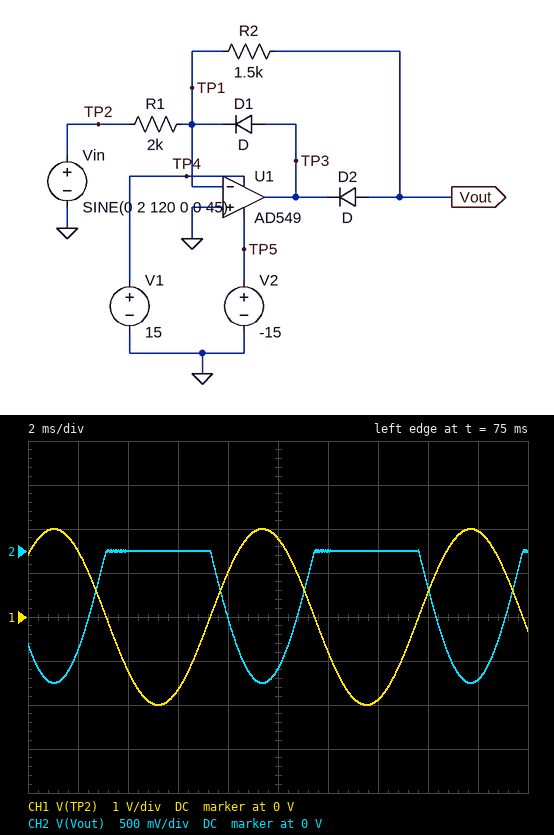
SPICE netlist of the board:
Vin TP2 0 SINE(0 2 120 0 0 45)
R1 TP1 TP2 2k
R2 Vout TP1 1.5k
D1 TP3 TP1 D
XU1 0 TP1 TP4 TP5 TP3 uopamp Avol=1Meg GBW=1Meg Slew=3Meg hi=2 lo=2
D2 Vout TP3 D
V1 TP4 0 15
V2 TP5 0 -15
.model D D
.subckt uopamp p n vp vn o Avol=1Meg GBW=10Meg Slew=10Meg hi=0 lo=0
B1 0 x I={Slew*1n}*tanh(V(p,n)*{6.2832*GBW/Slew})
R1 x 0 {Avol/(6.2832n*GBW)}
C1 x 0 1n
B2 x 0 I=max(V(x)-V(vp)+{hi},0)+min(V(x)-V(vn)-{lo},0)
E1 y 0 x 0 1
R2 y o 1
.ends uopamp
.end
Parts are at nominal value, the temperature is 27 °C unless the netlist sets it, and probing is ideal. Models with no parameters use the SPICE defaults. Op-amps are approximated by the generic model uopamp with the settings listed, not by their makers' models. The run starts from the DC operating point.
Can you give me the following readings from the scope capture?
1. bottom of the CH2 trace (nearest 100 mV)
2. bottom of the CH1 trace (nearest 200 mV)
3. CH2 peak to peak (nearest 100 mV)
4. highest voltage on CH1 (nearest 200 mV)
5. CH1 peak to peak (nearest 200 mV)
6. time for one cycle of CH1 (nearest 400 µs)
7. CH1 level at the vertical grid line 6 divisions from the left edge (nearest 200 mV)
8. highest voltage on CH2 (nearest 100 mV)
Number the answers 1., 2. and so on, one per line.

1. -1.5 V
2. -2.0 V
3. 1.5 V
4. 2.0 V
5. 4.0 V
6. 8.4 ms
7. -800 mV
8. 0 V
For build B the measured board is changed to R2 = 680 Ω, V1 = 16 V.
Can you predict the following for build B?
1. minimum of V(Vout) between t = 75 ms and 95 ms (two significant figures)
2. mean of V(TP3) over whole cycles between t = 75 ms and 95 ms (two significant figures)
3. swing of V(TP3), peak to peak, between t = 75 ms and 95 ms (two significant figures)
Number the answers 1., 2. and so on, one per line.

1. -680 mV
2. -220 mV
3. 2.0 V
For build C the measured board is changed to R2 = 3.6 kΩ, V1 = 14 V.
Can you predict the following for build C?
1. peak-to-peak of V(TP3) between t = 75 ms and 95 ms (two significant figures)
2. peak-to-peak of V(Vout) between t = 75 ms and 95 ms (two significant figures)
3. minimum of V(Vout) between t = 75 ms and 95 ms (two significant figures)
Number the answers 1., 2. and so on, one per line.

1. 4.9 V
2. 3.6 V
3. -3.6 V
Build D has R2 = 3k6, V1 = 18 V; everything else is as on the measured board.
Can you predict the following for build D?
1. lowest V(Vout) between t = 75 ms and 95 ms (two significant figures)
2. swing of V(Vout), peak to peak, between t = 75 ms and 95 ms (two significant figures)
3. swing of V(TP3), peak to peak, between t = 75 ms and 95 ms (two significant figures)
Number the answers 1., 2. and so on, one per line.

1. -3.6 V
2. 3.6 V
3. 4.9 V
